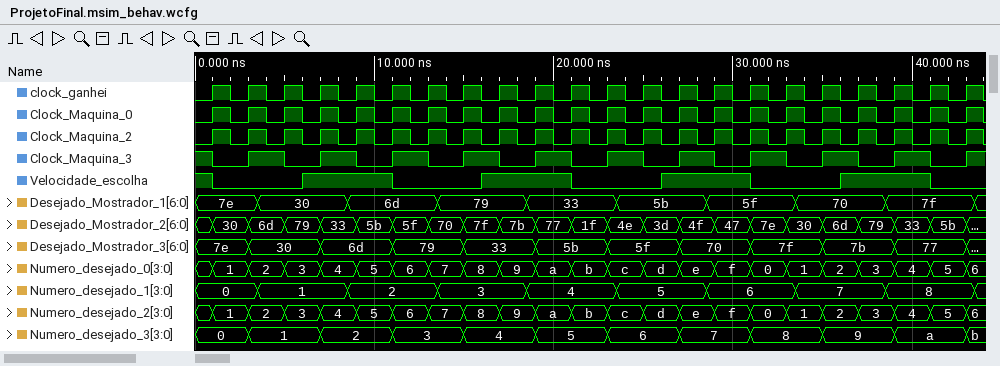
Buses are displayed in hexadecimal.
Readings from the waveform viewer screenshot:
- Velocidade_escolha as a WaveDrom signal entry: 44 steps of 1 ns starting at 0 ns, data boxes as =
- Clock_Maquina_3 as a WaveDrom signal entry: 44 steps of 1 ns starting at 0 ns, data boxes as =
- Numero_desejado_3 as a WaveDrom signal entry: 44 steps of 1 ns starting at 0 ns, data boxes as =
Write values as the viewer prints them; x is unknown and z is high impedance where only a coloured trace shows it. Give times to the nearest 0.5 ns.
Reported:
{name: 'Velocidade_escolha', wave: '10....1....0....1....0....1....0....1....0..'}
{name: 'Clock_Maquina_3', wave: '10.1.0.1.0.1.0.1.0.1.0.1.0.1.0.1.0.1.0.1.0.1'}
{name: 'Numero_desejado_3', wave: '=..=...=...=...=...=...=...=...=...=...=...=', data: '0 1 2 3 4 5 6 7 8 9 a b'}
